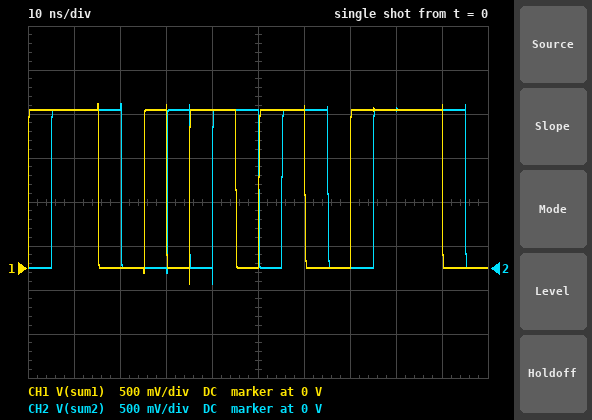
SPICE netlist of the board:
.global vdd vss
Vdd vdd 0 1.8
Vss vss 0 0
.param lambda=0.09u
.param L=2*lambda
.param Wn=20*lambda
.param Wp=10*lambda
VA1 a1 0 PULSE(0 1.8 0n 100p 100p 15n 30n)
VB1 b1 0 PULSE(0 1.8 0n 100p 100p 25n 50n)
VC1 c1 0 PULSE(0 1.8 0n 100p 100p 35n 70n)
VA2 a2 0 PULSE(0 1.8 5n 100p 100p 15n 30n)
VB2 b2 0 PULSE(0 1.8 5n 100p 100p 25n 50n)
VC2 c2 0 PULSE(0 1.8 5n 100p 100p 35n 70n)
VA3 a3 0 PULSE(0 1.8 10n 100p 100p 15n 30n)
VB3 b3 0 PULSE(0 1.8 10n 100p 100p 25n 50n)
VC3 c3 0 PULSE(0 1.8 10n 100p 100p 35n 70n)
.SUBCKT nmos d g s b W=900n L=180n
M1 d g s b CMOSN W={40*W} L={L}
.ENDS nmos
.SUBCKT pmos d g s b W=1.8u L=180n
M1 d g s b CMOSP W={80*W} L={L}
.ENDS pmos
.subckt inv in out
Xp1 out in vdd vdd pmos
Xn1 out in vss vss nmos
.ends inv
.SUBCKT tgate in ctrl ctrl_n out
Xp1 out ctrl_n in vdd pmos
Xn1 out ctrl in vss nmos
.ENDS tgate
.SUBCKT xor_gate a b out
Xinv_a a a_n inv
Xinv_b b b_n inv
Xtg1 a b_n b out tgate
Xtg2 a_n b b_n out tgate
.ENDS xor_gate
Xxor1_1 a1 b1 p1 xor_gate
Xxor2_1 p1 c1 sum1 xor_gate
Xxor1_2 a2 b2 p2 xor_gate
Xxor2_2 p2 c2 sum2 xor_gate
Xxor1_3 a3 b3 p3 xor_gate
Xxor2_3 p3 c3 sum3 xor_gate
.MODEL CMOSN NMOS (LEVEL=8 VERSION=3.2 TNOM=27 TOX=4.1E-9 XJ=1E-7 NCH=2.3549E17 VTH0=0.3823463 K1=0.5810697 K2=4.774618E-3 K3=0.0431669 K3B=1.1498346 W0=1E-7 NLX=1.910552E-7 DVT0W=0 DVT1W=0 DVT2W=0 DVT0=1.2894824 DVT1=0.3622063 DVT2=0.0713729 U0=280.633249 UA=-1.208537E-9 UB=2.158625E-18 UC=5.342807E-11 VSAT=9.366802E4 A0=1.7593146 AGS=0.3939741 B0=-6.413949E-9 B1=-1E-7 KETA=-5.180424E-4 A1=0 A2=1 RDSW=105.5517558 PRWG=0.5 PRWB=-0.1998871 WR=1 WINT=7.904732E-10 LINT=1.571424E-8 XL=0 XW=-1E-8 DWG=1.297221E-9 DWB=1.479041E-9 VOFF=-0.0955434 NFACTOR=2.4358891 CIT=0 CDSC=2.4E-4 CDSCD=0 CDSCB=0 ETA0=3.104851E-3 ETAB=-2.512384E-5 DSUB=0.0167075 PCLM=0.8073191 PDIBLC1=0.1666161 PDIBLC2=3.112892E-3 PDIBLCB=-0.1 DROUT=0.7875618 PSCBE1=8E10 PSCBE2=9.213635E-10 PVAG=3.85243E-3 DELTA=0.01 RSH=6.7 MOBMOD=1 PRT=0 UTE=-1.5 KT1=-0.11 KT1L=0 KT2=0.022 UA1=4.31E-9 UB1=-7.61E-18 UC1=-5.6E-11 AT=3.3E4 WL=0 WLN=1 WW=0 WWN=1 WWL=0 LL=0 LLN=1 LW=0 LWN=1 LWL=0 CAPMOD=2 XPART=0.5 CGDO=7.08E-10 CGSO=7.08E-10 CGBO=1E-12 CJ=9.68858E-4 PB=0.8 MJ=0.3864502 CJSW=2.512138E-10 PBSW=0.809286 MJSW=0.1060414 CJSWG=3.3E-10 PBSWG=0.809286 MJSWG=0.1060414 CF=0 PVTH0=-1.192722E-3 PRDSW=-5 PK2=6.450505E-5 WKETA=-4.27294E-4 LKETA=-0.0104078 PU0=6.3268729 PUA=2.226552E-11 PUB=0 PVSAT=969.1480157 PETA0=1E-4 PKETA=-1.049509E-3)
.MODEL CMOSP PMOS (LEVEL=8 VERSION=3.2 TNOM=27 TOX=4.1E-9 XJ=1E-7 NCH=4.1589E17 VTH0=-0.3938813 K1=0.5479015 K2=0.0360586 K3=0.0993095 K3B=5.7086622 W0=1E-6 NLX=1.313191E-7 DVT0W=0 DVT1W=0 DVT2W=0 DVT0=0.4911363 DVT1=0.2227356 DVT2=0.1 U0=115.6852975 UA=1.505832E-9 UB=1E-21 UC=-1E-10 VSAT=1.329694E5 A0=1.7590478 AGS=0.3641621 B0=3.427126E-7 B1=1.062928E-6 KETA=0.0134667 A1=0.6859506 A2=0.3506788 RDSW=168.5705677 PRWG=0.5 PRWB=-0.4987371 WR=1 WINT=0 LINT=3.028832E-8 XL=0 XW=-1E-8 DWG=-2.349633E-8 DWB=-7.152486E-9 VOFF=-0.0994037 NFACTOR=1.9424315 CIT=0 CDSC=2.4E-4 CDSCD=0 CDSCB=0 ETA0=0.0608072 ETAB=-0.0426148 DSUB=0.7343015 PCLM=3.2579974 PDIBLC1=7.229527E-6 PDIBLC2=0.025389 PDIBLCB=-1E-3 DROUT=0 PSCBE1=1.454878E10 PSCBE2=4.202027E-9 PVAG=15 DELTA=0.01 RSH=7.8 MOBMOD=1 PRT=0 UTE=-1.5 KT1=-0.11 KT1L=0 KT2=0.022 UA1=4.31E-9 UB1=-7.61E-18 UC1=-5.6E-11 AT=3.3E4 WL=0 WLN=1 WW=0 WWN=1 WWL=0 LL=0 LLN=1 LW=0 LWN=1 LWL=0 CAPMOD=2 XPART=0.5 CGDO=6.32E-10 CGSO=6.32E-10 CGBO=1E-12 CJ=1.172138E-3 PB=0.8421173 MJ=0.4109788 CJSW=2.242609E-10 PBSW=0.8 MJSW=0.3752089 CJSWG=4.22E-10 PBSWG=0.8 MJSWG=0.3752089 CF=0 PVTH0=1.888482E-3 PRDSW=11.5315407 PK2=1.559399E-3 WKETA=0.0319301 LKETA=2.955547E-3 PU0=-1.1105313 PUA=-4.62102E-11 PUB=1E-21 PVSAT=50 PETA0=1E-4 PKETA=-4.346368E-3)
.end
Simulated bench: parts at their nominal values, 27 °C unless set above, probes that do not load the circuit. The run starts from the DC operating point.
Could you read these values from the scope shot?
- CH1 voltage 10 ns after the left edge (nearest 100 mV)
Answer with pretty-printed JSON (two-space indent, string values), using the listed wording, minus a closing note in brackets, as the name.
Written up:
{
  "CH1 voltage 10 ns after the left edge": "1.8 V"
}
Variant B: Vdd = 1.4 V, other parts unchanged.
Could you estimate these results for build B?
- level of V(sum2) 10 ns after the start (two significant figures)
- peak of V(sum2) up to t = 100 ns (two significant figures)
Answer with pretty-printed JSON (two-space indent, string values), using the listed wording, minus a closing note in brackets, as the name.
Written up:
{
  "level of V(sum2) 10 ns after the start": "1.4 V",
  "peak of V(sum2) up to t = 100 ns": "1.8 V"
}
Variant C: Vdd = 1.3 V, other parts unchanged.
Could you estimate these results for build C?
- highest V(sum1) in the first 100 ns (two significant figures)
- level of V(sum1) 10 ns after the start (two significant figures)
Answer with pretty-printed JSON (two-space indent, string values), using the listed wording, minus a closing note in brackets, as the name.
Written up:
{
  "highest V(sum1) in the first 100 ns": "1.8 V",
  "level of V(sum1) 10 ns after the start": "1.3 V"
}
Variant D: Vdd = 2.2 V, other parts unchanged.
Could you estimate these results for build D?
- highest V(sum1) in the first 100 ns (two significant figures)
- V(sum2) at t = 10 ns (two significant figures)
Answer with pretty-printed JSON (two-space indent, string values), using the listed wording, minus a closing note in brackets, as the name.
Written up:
{
  "highest V(sum1) in the first 100 ns": "2.3 V",
  "V(sum2) at t = 10 ns": "2.2 V"
}
